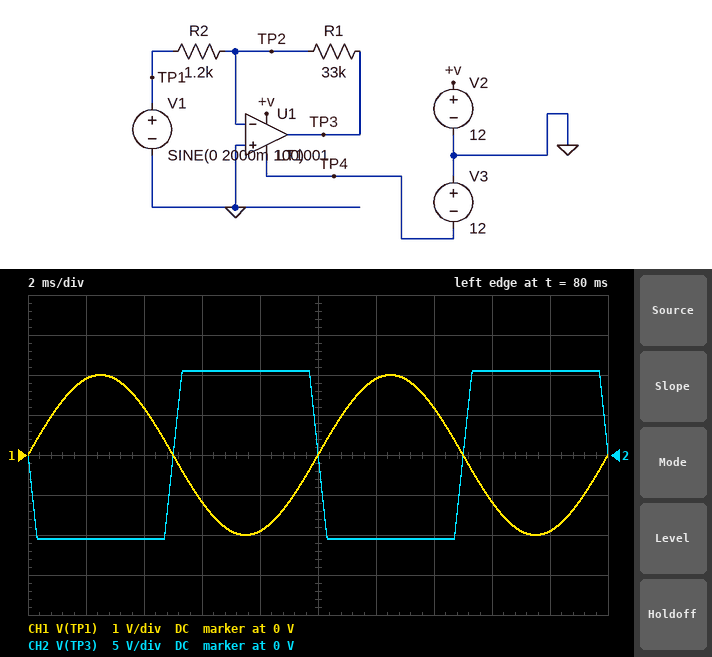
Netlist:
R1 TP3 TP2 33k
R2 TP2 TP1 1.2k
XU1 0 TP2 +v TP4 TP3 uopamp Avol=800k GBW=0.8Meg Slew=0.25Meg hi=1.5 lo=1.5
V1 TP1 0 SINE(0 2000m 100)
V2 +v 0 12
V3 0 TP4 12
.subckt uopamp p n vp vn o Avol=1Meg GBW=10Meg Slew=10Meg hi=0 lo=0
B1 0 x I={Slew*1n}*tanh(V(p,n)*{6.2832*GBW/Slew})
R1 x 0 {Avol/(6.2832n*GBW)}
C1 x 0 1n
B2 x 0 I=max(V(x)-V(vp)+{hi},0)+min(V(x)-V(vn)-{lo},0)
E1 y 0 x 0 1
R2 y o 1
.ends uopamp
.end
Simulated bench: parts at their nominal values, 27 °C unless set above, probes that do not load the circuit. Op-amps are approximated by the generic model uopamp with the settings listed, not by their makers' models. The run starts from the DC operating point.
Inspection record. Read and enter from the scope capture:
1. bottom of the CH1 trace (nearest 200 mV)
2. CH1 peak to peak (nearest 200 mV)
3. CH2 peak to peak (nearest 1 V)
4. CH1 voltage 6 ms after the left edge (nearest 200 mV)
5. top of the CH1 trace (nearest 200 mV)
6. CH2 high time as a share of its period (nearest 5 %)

-2.0 V
4.0 V
21 V
-1.2 V
2.0 V
50 %
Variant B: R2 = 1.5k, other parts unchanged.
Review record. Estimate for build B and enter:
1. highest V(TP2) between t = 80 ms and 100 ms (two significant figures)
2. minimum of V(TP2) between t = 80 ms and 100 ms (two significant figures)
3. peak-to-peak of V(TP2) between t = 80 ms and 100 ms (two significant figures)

1.5 V
-1.5 V
2.9 V
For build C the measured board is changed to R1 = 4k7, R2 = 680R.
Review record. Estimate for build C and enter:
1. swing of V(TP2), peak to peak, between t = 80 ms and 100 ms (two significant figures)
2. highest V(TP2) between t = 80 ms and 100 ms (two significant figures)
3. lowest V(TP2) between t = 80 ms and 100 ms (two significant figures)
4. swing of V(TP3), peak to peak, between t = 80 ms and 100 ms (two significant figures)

840 mV
420 mV
-420 mV
21 V
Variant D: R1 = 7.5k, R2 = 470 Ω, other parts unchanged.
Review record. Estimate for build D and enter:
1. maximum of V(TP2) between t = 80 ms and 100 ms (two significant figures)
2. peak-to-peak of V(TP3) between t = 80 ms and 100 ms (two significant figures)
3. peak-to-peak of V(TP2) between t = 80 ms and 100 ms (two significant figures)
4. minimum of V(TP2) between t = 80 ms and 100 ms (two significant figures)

1.3 V
21 V
2.5 V
-1.3 V
